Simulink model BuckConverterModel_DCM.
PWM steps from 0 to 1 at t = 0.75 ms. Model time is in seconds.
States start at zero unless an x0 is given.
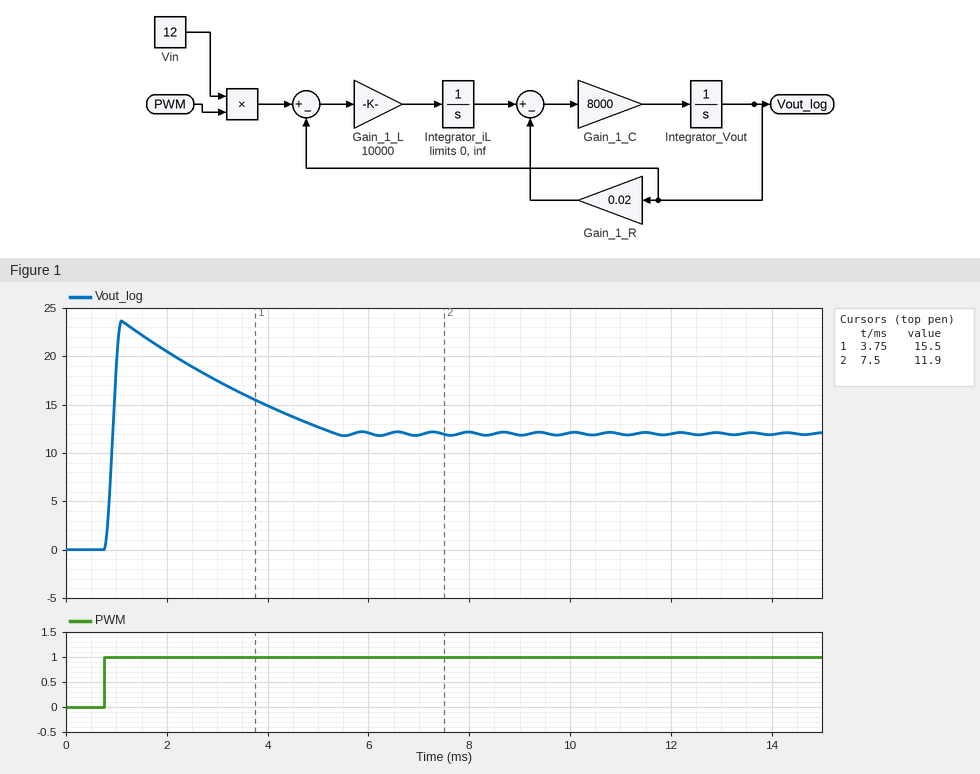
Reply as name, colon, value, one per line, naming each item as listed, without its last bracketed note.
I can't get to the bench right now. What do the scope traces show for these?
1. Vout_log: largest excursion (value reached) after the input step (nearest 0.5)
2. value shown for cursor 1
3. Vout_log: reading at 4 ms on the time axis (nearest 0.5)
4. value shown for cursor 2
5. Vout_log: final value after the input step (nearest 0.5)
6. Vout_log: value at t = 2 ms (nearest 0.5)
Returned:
Vout_log: largest excursion (value reached) after the input step: 23.5
value shown for cursor 1: 15.5
Vout_log: reading at 4 ms on the time axis: 15.0
value shown for cursor 2: 11.9
Vout_log: final value after the input step: 12.0
Vout_log: value at t = 2 ms: 20.5
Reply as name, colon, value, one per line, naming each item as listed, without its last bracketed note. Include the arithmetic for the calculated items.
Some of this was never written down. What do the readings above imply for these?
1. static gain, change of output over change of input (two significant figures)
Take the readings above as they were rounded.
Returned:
static gain, change of output over change of input: (12 - 0) / (1 - 0) = 12
